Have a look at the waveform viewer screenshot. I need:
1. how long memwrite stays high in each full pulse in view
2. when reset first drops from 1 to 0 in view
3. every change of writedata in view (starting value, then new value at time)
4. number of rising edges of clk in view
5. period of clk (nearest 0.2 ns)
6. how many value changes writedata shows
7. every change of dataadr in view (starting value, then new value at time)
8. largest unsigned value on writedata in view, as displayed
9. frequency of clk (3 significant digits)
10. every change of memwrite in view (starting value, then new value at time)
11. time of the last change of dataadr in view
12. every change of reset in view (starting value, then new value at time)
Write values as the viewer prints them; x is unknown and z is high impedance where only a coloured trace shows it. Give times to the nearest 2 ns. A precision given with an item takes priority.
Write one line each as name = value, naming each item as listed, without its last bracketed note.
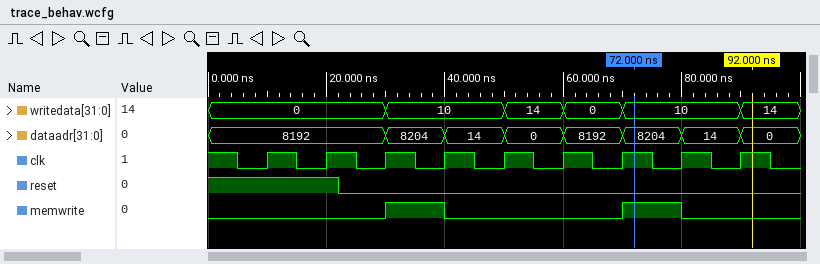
how long memwrite stays high in each full pulse in view = 10 ns, 10 ns
when reset first drops from 1 to 0 in view = 22 ns
every change of writedata in view = 0, 10 at 30 ns, 14 at 50 ns, 0 at 60 ns, 10 at 70 ns, 14 at 90 ns
number of rising edges of clk in view = 9
period of clk = 10 ns
how many value changes writedata shows = 5
every change of dataadr in view = 8192, 8204 at 30 ns, 14 at 40 ns, 0 at 50 ns, 8192 at 60 ns, 8204 at 70 ns, 14 at 80 ns, 0 at 90 ns
largest unsigned value on writedata in view, as displayed = 14
frequency of clk = 100 MHz
every change of memwrite in view = 0, 1 at 30 ns, 0 at 40 ns, 1 at 70 ns, 0 at 80 ns
time of the last change of dataadr in view = 90 ns
every change of reset in view = 1, 0 at 22 ns
